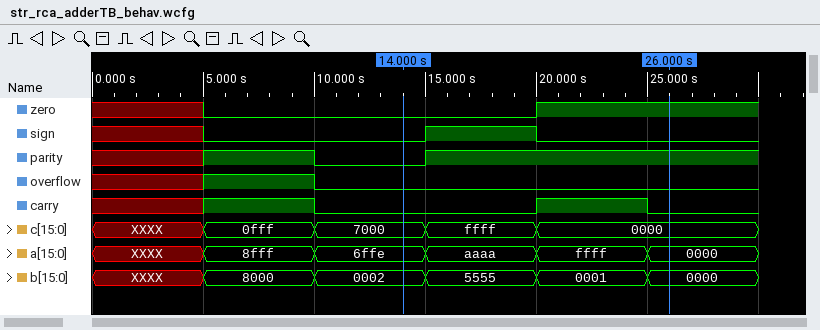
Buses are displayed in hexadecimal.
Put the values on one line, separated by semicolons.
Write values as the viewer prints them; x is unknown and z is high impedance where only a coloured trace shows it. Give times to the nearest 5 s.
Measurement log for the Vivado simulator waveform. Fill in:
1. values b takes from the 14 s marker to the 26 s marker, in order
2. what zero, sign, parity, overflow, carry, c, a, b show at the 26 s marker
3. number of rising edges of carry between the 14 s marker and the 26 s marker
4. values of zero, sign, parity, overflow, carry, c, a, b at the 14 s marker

0002, 5555, 0001, 0000; zero=1, sign=0, parity=1, overflow=0, carry=0, c=0000, a=0000, b=0000; 1; zero=0, sign=0, parity=0, overflow=0, carry=0, c=7000, a=6ffe, b=0002
